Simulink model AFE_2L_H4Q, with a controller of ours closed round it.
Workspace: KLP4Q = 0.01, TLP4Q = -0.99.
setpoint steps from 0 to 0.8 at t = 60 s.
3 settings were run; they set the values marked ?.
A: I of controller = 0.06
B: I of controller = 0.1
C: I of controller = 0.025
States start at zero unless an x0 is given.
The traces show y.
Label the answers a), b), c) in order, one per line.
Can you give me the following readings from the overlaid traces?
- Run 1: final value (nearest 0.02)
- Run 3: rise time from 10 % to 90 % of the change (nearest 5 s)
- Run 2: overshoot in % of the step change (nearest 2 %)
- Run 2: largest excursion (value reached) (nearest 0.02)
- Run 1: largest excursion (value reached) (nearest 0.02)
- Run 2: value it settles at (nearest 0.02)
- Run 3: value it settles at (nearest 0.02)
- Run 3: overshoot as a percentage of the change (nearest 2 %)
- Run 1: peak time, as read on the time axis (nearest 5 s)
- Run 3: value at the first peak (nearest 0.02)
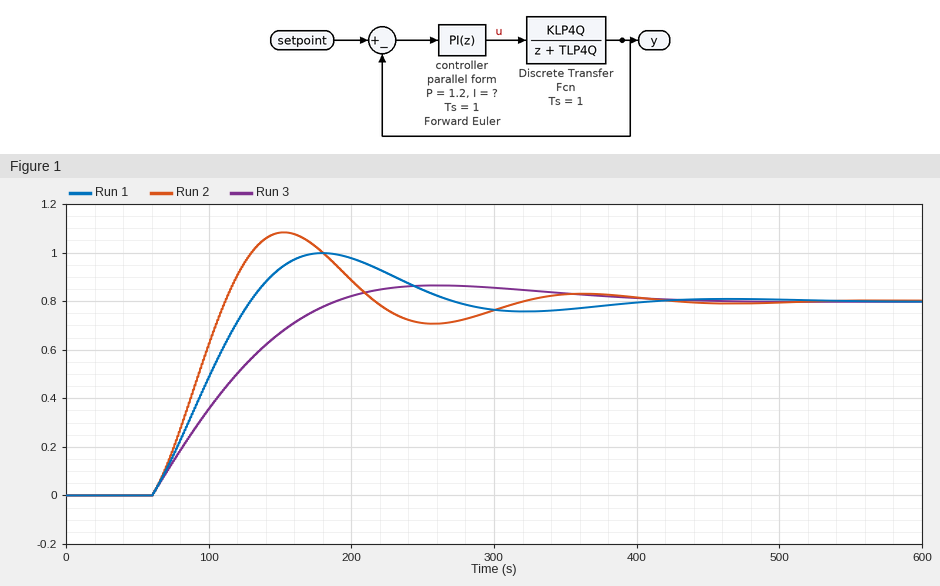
a) 0.80
b) 95 s
c) 36 %
d) 1.08
e) 1.00
f) 0.80
g) 0.80
h) 8 %
i) 180 s
j) 0.86
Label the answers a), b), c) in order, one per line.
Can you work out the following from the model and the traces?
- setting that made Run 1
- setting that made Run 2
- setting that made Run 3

a) A
b) B
c) C
